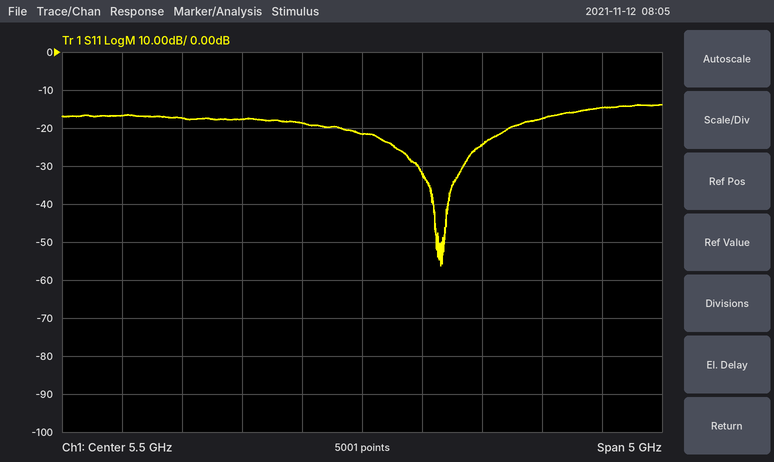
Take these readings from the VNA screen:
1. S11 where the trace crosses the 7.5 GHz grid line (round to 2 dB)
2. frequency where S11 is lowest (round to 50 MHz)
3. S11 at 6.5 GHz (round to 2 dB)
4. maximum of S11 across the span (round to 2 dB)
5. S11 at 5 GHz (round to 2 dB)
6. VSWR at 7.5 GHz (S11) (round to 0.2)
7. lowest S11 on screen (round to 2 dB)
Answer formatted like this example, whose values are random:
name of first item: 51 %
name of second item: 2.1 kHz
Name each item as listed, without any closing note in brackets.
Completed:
S11 where the trace crosses the 7.5 GHz grid line: -14 dB
frequency where S11 is lowest: 6.15 GHz
S11 at 6.5 GHz: -24 dB
maximum of S11 across the span: -14 dB
S11 at 5 GHz: -18 dB
VSWR at 7.5 GHz (S11): 1.4
lowest S11 on screen: -56 dB
